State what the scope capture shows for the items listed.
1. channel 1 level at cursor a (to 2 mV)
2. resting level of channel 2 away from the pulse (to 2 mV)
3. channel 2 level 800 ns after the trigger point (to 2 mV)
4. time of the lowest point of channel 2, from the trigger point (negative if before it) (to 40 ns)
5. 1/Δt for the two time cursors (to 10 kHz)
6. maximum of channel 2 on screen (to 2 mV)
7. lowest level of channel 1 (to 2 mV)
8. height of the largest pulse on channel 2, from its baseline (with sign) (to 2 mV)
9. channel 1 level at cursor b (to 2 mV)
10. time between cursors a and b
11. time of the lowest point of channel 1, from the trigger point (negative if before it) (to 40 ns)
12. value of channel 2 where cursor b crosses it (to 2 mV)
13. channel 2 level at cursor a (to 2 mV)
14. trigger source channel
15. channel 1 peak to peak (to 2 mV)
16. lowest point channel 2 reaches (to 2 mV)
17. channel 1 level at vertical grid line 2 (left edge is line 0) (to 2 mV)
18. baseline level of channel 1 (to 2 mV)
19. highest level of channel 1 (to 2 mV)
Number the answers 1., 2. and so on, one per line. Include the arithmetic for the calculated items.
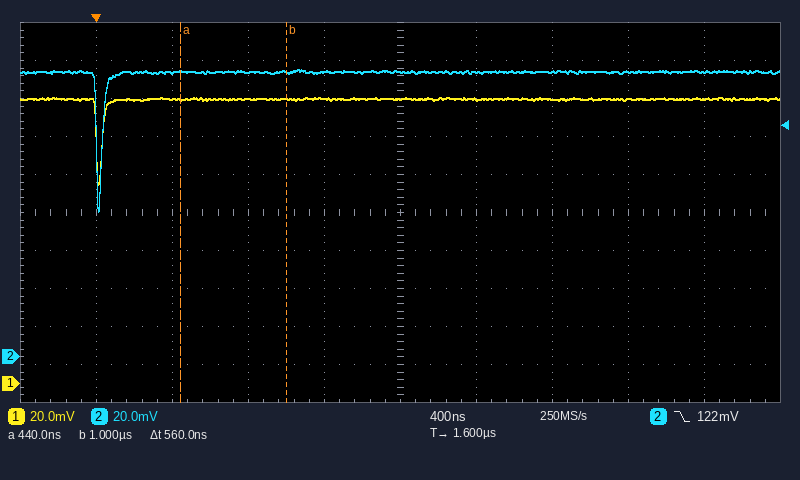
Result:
1. 150 mV
2. 150 mV
3. 150 mV
4. 0 ns
5. 1 / 560 ns ≈ 1.79 MHz
6. 152 mV
7. 104 mV
8. 76 mV − (150 mV) = -74 mV
9. 150 mV
10. 560 ns
11. 0 ns
12. 150 mV
13. 150 mV
14. channel 2
15. 150 mV − (104 mV) = 46 mV
16. 76 mV
17. 150 mV
18. 150 mV
19. 150 mV
